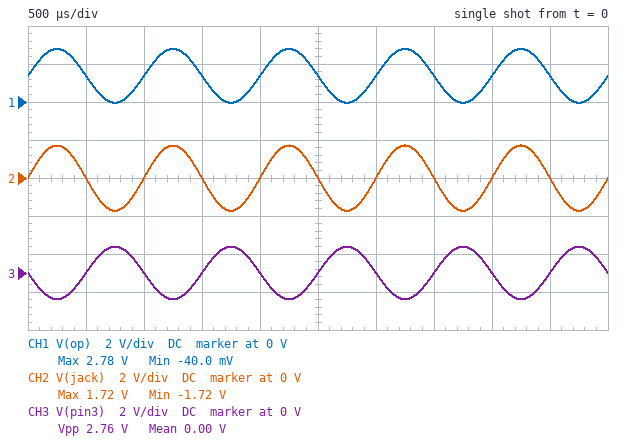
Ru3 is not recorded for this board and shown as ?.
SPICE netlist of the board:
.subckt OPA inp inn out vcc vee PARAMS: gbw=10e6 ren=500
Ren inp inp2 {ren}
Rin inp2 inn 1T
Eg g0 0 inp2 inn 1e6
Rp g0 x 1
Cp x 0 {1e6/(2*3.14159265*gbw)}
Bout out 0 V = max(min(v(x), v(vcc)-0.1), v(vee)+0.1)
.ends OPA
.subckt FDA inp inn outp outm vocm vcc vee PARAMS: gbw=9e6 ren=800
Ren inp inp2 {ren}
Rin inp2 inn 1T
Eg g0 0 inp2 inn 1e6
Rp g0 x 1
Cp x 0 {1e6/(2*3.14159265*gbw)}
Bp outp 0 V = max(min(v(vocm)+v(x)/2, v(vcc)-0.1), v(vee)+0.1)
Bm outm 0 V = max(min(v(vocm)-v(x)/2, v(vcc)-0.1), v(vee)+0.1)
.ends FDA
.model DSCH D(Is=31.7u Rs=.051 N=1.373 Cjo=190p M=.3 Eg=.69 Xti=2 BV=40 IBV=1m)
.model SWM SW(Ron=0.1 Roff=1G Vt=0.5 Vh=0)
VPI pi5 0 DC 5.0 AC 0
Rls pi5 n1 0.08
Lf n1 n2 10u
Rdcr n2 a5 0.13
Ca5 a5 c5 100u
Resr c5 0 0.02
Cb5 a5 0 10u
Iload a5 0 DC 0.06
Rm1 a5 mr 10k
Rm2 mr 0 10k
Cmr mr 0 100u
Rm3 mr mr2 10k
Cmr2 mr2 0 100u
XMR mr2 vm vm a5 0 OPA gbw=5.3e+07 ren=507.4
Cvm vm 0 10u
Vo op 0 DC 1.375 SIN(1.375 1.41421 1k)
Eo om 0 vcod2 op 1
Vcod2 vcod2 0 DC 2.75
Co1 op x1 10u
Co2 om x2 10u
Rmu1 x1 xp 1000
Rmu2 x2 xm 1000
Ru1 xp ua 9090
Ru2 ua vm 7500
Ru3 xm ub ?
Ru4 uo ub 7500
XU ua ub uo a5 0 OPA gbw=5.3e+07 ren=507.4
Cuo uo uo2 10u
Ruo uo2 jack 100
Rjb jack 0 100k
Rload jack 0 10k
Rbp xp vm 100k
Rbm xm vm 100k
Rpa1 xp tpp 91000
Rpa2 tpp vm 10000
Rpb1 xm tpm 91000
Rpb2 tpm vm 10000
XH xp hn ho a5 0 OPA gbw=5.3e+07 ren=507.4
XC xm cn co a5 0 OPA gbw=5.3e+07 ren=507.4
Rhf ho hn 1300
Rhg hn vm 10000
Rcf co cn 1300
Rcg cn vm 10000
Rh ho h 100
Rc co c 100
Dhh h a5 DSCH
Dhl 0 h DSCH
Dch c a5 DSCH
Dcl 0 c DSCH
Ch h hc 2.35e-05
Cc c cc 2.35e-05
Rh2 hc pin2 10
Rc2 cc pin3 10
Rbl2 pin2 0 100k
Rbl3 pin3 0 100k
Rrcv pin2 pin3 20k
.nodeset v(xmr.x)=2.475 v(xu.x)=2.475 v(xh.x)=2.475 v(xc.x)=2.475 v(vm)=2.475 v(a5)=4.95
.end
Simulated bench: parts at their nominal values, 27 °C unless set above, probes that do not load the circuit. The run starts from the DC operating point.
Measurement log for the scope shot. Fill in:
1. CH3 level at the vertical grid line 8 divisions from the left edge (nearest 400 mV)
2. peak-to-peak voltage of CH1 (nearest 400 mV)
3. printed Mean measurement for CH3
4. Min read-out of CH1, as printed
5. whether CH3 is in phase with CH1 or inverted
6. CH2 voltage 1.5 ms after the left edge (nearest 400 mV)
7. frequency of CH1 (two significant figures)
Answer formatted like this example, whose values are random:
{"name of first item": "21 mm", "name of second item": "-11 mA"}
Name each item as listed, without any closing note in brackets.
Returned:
{"CH3 level at the vertical grid line 8 divisions from the left edge": "0 V", "peak-to-peak voltage of CH1": "2.8 V", "printed Mean measurement for CH3": "0.00 V", "Min read-out of CH1, as printed": "-40.0 mV", "whether CH3 is in phase with CH1 or inverted": "inverted", "CH2 voltage 1.5 ms after the left edge": "0 V", "frequency of CH1": "1.0 kHz"}
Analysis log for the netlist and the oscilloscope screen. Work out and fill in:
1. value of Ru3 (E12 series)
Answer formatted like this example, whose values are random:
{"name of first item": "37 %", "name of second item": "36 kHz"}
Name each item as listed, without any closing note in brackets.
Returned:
{"value of Ru3": "12 kΩ"}
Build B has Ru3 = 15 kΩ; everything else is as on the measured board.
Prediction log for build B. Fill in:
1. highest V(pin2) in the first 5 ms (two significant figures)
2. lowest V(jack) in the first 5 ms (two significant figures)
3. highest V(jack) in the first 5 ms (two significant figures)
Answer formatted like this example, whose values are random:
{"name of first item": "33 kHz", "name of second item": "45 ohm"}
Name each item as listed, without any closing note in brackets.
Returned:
{"highest V(pin2) in the first 5 ms": "1.5 V", "lowest V(jack) in the first 5 ms": "-1.5 V", "highest V(jack) in the first 5 ms": "1.5 V"}
